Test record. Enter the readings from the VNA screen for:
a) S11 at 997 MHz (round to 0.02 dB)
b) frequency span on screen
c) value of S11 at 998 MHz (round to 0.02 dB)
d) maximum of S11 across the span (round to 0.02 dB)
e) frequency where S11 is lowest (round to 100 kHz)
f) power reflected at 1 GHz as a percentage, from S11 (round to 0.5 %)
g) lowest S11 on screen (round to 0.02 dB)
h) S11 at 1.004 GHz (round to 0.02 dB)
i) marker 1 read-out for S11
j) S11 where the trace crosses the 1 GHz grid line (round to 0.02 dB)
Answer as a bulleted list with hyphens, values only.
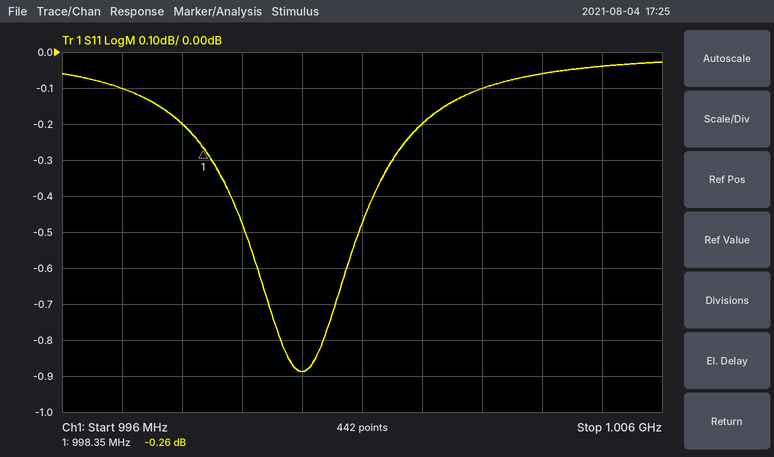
- -0.10 dB
- 10 MHz
- -0.20 dB
- -0.02 dB
- 1.0000 GHz
- 81.5 %
- -0.88 dB
- -0.06 dB
- -0.26 dB
- -0.88 dB
